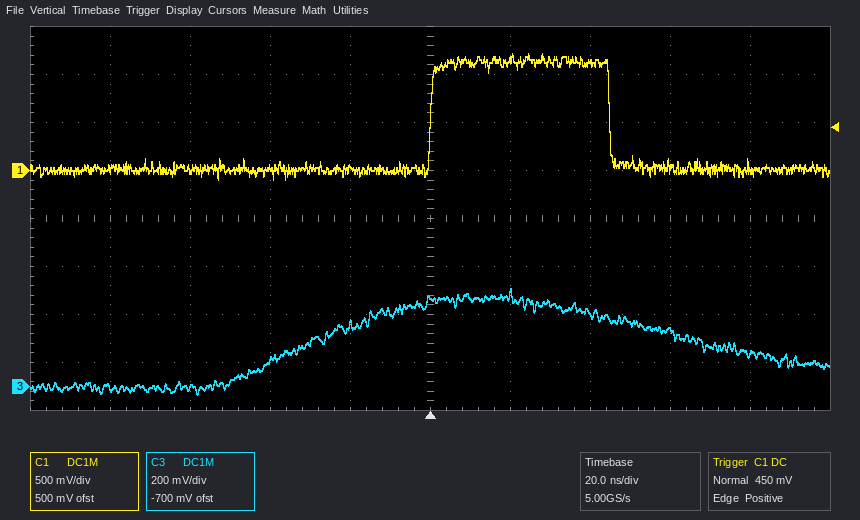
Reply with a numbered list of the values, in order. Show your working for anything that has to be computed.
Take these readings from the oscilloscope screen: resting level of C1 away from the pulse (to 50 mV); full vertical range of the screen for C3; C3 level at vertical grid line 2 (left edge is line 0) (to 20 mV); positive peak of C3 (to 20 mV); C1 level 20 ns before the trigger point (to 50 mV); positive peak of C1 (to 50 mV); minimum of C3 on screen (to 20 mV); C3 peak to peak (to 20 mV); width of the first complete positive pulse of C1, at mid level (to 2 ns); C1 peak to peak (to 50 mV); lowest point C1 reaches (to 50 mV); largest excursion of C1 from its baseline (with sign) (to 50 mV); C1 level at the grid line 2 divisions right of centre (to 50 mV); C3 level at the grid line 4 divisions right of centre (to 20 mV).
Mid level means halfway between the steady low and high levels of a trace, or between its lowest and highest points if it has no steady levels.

1. 0 mV
2. 1.6 V
3. 0 mV
4. 400 mV
5. 0 mV
6. 1.20 V
7. -40 mV
8. 400 mV − (-40 mV) = 440 mV
9. 44 ns
10. 1.20 V − (-100 mV) = 1.30 V
11. -100 mV
12. 1.20 V − (0 mV) = +1.20 V
13. 1.10 V
14. 140 mV
